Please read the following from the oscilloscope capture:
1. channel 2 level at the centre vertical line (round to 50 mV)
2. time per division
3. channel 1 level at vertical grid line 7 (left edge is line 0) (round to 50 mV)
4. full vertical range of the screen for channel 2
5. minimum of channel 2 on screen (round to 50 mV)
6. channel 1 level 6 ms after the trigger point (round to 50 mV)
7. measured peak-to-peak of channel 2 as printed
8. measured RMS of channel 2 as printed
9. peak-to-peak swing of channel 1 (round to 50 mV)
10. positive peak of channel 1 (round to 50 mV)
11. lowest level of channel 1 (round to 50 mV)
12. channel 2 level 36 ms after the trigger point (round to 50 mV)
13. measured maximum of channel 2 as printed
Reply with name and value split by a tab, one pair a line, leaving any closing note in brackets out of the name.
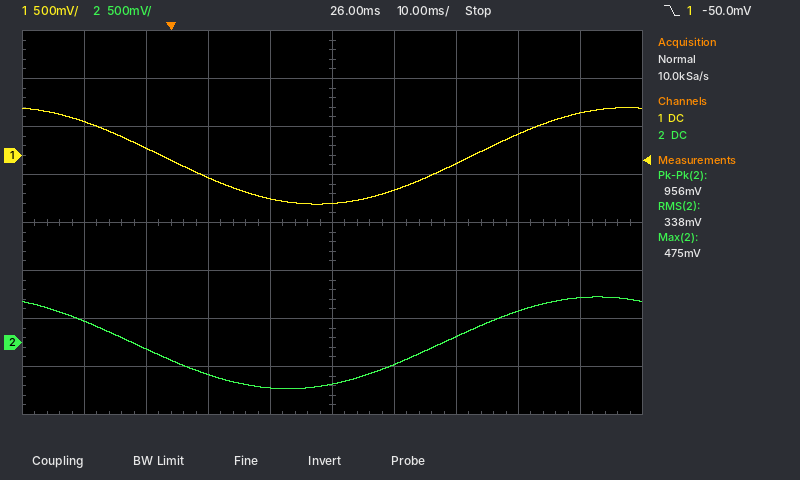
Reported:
channel 2 level at the centre vertical line	-450 mV
time per division	10 ms
channel 1 level at vertical grid line 7 (left edge is line 0)	-100 mV
full vertical range of the screen for channel 2	4 V
minimum of channel 2 on screen	-500 mV
channel 1 level 6 ms after the trigger point	-250 mV
measured peak-to-peak of channel 2 as printed	956 mV
measured RMS of channel 2 as printed	338 mV
peak-to-peak swing of channel 1	1.00 V
positive peak of channel 1	500 mV
lowest level of channel 1	-500 mV
channel 2 level 36 ms after the trigger point	-250 mV
measured maximum of channel 2 as printed	475 mV
